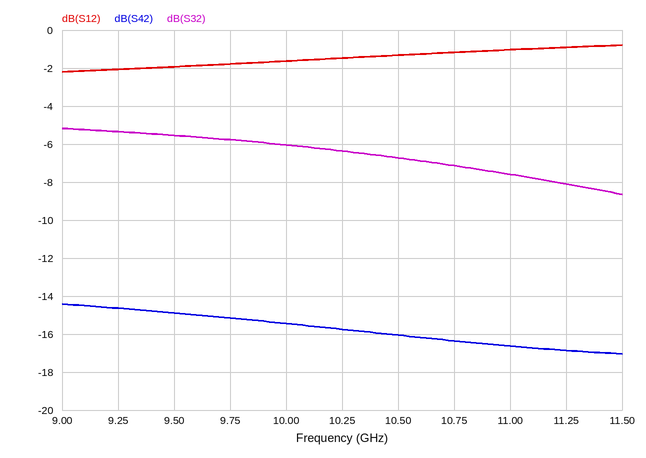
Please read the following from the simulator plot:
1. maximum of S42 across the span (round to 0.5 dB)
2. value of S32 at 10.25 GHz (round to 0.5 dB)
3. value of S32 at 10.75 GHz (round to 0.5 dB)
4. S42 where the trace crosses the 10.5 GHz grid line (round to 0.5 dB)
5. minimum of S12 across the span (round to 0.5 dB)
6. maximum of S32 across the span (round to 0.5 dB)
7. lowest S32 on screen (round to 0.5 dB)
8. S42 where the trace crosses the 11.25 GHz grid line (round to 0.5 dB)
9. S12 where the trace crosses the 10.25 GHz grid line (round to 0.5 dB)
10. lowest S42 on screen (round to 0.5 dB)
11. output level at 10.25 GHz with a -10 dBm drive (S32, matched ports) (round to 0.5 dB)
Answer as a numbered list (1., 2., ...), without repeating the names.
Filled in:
1. -14.5 dB
2. -6.5 dB
3. -7.0 dB
4. -16.0 dB
5. -2.0 dB
6. -5.0 dB
7. -8.5 dB
8. -17.0 dB
9. -1.5 dB
10. -17.0 dB
11. -16.5 dBm
